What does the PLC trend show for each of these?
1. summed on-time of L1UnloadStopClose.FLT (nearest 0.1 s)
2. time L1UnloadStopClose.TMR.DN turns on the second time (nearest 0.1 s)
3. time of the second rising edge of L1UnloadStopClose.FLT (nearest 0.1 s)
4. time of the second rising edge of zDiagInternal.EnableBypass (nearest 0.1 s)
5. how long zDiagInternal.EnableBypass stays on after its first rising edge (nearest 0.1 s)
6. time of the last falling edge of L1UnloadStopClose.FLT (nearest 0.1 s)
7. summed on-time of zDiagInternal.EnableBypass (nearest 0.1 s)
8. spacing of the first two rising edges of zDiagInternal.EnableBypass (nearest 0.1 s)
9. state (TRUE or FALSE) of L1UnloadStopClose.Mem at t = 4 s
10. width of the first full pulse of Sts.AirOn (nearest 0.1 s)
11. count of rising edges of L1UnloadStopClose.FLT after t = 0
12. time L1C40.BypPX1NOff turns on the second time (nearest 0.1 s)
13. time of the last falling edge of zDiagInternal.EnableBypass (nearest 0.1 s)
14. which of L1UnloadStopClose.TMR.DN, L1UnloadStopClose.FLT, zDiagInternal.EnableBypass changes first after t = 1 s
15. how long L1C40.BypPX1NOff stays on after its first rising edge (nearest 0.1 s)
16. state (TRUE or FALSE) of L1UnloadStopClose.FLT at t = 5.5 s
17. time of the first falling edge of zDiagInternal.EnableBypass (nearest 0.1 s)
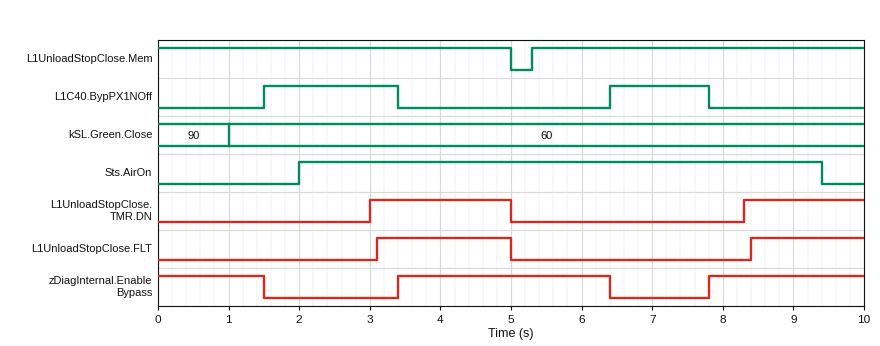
3.5 s
8.3 s
8.4 s
7.8 s
3.0 s
5.0 s
6.7 s
4.4 s
TRUE
7.4 s
2
6.4 s
6.4 s
zDiagInternal.EnableBypass
1.9 s
FALSE
1.5 s
